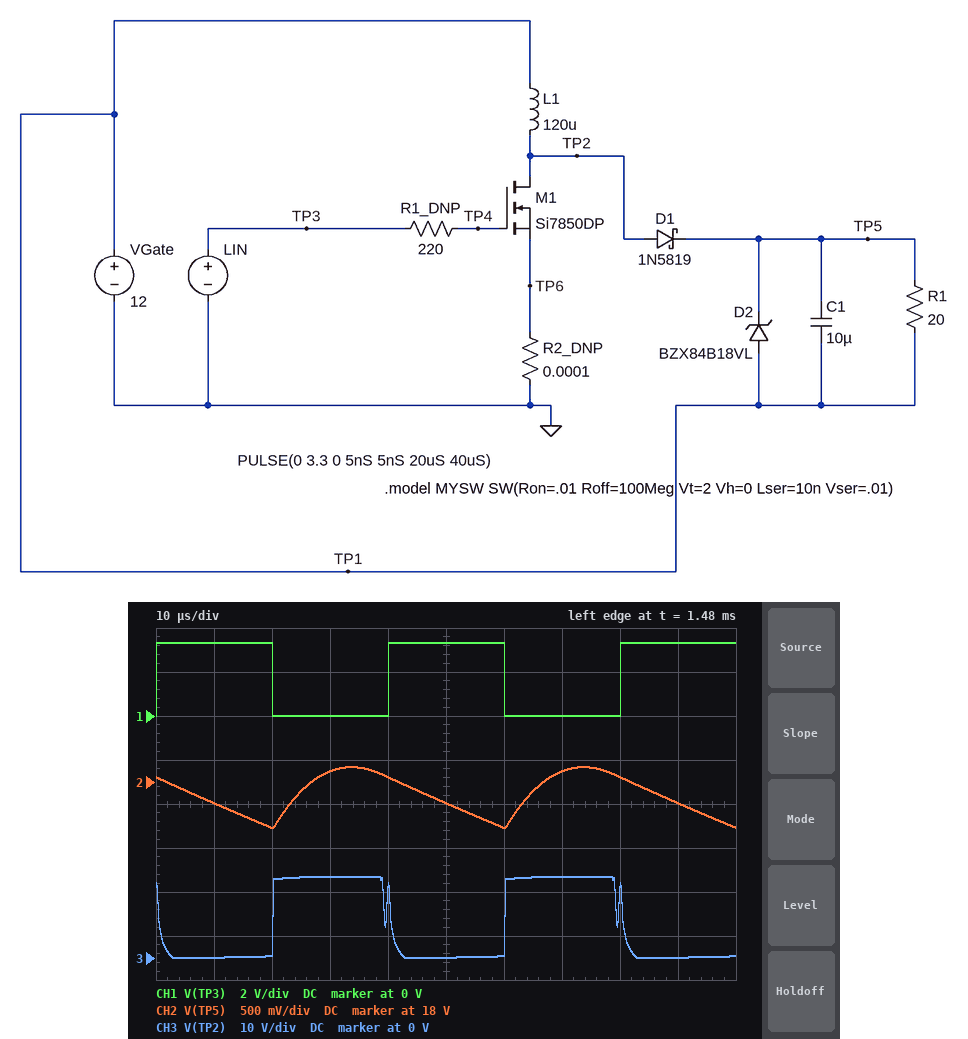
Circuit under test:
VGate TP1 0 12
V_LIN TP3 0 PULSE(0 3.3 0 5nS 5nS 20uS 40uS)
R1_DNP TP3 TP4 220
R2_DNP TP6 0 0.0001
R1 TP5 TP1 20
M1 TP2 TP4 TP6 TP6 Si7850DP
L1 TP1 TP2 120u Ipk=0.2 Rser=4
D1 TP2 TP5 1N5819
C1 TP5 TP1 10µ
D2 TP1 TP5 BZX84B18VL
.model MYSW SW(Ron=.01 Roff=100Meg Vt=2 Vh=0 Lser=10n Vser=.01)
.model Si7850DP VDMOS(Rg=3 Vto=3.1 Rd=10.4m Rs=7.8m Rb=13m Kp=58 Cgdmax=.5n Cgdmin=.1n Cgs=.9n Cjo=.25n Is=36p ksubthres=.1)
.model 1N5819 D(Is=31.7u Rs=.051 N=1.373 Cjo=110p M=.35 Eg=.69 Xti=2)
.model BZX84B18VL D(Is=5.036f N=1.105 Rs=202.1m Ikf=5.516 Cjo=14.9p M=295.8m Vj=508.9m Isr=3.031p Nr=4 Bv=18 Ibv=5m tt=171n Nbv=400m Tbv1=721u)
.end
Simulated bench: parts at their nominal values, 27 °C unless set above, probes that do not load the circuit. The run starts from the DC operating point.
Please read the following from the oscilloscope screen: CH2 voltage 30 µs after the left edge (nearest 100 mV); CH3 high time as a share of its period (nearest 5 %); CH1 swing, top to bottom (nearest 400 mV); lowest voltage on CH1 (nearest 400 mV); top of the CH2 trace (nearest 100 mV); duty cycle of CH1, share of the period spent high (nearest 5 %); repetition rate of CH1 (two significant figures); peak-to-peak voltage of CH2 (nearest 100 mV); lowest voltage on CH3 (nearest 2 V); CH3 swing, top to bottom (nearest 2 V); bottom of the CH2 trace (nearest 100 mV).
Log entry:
18.1 V
50 %
3.2 V
0 V
18.2 V
50 %
25 kHz
700 mV
0 V
18 V
17.5 V
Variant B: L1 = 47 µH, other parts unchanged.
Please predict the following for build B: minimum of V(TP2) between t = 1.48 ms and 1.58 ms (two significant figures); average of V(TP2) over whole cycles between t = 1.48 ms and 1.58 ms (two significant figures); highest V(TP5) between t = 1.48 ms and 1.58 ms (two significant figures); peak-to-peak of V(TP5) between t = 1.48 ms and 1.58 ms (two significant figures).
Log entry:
110 mV
8.7 V
16 V
590 mV
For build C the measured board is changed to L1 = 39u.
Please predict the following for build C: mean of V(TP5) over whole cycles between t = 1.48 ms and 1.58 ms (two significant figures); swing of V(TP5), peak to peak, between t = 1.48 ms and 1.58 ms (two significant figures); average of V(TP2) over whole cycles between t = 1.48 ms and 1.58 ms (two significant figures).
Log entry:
15 V
450 mV
8.8 V
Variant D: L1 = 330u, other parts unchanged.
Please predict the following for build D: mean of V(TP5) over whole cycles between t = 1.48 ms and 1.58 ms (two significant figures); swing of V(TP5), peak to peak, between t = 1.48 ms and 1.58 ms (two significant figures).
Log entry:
17 V
520 mV
